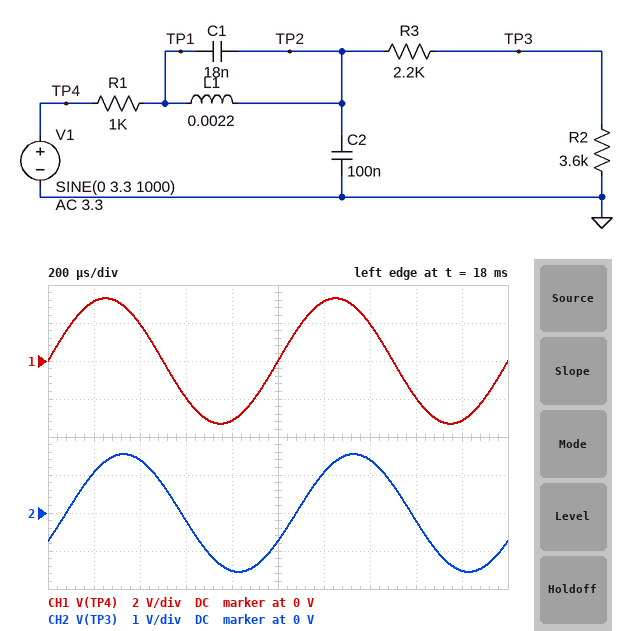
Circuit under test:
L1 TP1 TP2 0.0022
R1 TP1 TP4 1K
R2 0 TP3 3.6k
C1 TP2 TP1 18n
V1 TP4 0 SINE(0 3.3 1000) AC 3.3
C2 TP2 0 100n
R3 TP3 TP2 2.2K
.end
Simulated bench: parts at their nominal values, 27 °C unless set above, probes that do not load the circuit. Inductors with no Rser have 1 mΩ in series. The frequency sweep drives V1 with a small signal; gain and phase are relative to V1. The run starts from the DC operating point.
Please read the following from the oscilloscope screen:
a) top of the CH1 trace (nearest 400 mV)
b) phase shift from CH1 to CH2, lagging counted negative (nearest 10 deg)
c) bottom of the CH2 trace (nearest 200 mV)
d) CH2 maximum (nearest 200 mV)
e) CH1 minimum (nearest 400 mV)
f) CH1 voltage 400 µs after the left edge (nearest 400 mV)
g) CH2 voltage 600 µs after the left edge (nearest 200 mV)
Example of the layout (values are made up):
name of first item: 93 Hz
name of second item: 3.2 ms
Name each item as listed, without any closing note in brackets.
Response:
top of the CH1 trace: 3.2 V
phase shift from CH1 to CH2, lagging counted negative: -30 deg
bottom of the CH2 trace: -1.6 V
CH2 maximum: 1.6 V
CH1 minimum: -3.2 V
CH1 voltage 400 µs after the left edge: 2.0 V
CH2 voltage 600 µs after the left edge: -200 mV
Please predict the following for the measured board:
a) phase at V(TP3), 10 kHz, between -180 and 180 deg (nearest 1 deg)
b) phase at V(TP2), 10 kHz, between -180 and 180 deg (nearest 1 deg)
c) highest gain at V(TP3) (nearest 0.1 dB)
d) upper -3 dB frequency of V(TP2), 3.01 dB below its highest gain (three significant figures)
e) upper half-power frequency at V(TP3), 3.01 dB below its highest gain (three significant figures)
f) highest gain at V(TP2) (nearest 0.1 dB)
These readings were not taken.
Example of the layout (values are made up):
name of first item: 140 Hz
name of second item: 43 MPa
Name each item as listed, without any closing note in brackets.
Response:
phase at V(TP3), 10 kHz, between -180 and 180 deg: -89 deg
phase at V(TP2), 10 kHz, between -180 and 180 deg: -89 deg
highest gain at V(TP3): -5.5 dB
upper -3 dB frequency of V(TP2), 3.01 dB below its highest gain: 1.91 kHz
upper half-power frequency at V(TP3), 3.01 dB below its highest gain: 1.91 kHz
highest gain at V(TP2): -1.4 dB
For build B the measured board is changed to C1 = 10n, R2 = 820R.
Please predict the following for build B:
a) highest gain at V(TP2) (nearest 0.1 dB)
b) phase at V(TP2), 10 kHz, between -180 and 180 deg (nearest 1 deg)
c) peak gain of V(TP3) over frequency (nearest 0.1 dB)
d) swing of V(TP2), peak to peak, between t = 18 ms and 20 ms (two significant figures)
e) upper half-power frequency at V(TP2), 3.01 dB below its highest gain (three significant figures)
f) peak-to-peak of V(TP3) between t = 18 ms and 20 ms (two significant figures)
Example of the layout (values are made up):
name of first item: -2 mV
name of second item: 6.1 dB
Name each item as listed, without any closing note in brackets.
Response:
highest gain at V(TP2): -2.5 dB
phase at V(TP2), 10 kHz, between -180 and 180 deg: -87 deg
peak gain of V(TP3) over frequency: -13.8 dB
swing of V(TP2), peak to peak, between t = 18 ms and 20 ms: 4.5 V
upper half-power frequency at V(TP2), 3.01 dB below its highest gain: 2.17 kHz
peak-to-peak of V(TP3) between t = 18 ms and 20 ms: 1.2 V
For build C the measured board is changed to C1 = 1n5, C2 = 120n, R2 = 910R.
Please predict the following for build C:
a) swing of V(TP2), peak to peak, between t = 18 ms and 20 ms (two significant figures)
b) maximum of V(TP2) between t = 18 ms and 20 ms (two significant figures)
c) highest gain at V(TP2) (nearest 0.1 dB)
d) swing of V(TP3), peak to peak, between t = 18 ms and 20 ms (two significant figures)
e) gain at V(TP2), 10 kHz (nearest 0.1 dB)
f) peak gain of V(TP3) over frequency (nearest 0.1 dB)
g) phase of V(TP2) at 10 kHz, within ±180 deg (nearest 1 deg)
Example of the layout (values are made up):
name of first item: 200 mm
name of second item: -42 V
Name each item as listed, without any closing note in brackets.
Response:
swing of V(TP2), peak to peak, between t = 18 ms and 20 ms: 4.4 V
maximum of V(TP2) between t = 18 ms and 20 ms: 2.2 V
highest gain at V(TP2): -2.4 dB
swing of V(TP3), peak to peak, between t = 18 ms and 20 ms: 1.3 V
gain at V(TP2), 10 kHz: -17.6 dB
peak gain of V(TP3) over frequency: -13.1 dB
phase of V(TP2) at 10 kHz, within ±180 deg: -88 deg
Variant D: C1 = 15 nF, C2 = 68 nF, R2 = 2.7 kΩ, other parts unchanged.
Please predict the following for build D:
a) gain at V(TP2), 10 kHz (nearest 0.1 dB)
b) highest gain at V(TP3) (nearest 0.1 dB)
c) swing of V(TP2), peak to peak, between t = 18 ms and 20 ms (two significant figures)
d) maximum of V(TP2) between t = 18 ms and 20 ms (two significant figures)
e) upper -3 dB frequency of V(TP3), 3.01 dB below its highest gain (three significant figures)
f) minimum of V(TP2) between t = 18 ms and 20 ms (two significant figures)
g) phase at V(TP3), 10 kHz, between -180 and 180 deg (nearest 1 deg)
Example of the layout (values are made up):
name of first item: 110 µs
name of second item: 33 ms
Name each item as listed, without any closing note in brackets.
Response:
gain at V(TP2), 10 kHz: -12.7 dB
highest gain at V(TP3): -6.8 dB
swing of V(TP2), peak to peak, between t = 18 ms and 20 ms: 5.2 V
maximum of V(TP2) between t = 18 ms and 20 ms: 2.6 V
upper -3 dB frequency of V(TP3), 3.01 dB below its highest gain: 2.91 kHz
minimum of V(TP2) between t = 18 ms and 20 ms: -2.6 V
phase at V(TP3), 10 kHz, between -180 and 180 deg: -83 deg
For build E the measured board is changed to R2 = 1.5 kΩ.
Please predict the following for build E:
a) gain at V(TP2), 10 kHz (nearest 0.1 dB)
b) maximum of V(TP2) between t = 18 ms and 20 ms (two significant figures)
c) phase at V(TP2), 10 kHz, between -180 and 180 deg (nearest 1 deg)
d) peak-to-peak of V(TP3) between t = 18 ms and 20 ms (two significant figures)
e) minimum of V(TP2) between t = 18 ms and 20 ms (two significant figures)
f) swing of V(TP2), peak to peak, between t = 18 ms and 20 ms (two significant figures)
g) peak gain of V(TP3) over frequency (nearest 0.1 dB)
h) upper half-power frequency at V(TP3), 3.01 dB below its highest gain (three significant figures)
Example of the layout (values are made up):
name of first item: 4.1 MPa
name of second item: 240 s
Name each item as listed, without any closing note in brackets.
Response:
gain at V(TP2), 10 kHz: -16.0 dB
maximum of V(TP2) between t = 18 ms and 20 ms: 2.3 V
phase at V(TP2), 10 kHz, between -180 and 180 deg: -88 deg
peak-to-peak of V(TP3) between t = 18 ms and 20 ms: 1.9 V
minimum of V(TP2) between t = 18 ms and 20 ms: -2.3 V
swing of V(TP2), peak to peak, between t = 18 ms and 20 ms: 4.7 V
peak gain of V(TP3) over frequency: -9.9 dB
upper half-power frequency at V(TP3), 3.01 dB below its highest gain: 2.07 kHz
